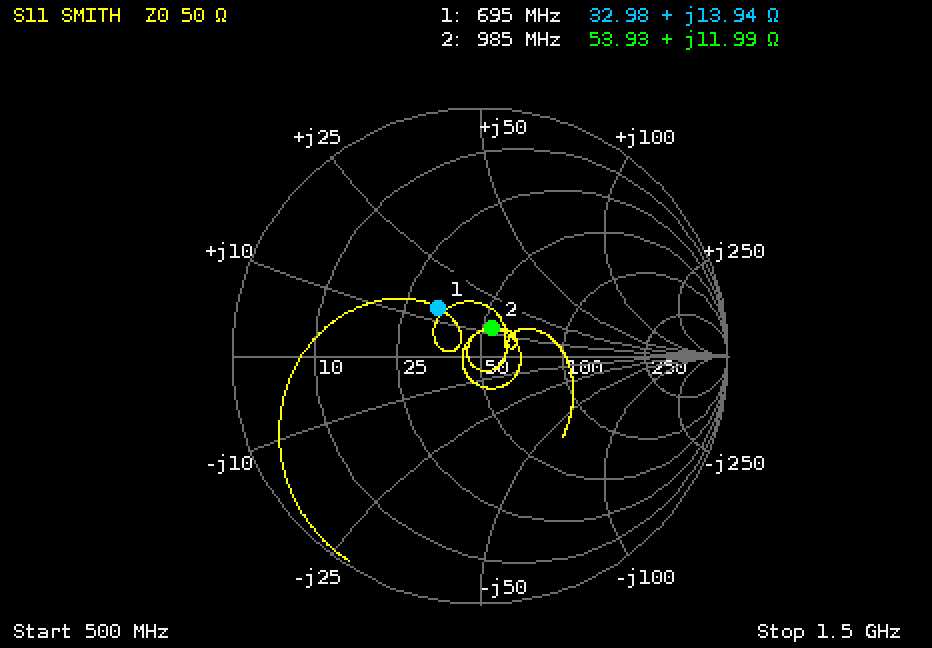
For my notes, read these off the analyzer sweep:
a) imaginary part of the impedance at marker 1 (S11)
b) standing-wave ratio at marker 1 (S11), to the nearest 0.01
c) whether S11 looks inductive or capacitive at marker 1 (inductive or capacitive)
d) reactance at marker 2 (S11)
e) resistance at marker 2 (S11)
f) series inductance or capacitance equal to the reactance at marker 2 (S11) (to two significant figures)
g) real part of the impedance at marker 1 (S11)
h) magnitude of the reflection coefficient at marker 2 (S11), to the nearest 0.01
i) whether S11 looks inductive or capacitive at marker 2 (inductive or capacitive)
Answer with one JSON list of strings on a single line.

["+13.94 Ω", "1.71", "inductive", "+11.99 Ω", "53.93 Ω", "1.9 nH", "32.98 Ω", "0.12", "inductive"]
